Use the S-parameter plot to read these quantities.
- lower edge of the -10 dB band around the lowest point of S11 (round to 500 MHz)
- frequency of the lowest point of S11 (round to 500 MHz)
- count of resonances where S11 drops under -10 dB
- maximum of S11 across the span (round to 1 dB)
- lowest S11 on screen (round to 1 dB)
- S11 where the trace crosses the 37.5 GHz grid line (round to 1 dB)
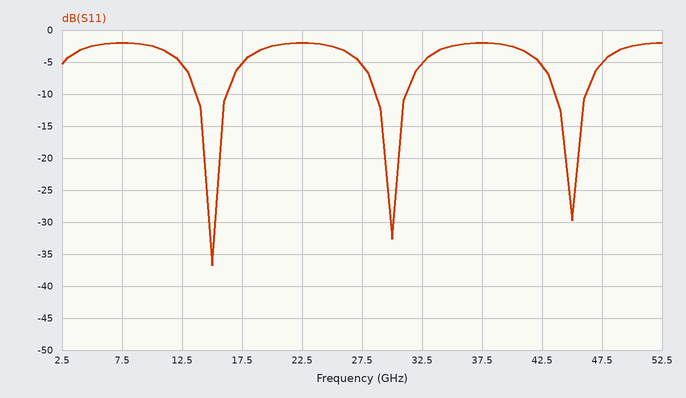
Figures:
13.5 GHz
15.0 GHz
3
-2 dB
-37 dB
-2 dB
